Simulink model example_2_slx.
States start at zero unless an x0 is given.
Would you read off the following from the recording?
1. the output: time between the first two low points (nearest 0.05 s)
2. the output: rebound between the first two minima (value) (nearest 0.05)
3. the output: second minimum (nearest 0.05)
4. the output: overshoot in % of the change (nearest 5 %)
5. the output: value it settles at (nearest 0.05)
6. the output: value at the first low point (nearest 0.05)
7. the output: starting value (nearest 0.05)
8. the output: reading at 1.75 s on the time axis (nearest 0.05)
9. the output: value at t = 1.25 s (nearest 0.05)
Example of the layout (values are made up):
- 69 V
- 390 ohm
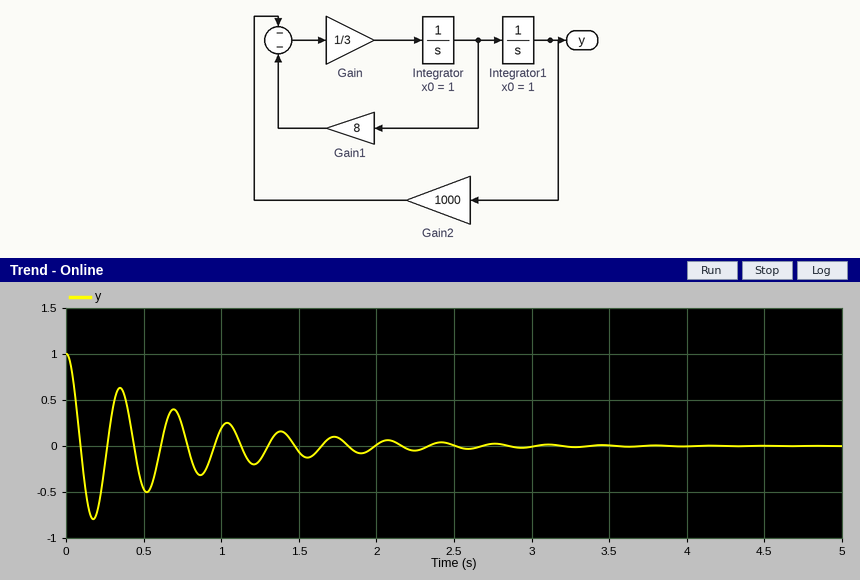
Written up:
- 0.35 s
- 0.65
- -0.50
- 80 %
- 0.00
- -0.80
- 1.00
- 0.10
- -0.15
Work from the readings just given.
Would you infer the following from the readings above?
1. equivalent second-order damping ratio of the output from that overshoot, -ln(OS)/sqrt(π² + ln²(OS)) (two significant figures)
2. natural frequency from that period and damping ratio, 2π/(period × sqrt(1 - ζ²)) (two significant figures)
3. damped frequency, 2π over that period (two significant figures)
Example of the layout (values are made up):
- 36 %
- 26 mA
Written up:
- 0.071
- 18 rad/s
- 18 rad/s
